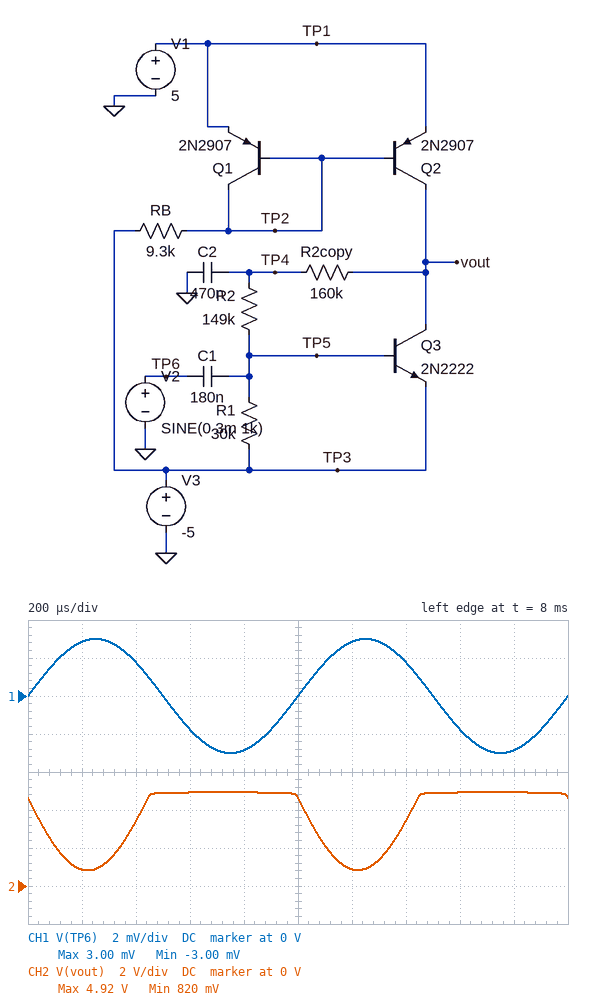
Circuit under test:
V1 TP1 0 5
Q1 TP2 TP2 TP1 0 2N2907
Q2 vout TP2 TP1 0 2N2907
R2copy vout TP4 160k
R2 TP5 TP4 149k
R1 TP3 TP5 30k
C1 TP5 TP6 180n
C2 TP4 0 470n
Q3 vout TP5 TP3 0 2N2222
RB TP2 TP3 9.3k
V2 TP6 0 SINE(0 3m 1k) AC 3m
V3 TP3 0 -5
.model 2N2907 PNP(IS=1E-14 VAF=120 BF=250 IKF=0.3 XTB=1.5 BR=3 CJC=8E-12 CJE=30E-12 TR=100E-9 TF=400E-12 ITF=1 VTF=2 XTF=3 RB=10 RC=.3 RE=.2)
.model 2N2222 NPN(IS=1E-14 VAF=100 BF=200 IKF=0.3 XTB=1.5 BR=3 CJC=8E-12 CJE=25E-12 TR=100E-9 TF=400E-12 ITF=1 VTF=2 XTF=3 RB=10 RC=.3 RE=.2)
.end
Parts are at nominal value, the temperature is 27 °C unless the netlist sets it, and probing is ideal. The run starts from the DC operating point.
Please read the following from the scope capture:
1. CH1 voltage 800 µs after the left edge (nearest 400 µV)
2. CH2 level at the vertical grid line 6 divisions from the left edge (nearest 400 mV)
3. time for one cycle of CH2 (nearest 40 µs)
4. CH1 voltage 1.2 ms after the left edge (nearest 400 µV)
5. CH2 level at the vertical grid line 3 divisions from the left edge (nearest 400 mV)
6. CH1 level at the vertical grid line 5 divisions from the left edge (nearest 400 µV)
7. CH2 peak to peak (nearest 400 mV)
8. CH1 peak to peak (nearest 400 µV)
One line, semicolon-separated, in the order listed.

-2.8 mV; 800 mV; 1.00 ms; 2.8 mV; 4.8 V; 0 V; 4.0 V; 6.0 mV
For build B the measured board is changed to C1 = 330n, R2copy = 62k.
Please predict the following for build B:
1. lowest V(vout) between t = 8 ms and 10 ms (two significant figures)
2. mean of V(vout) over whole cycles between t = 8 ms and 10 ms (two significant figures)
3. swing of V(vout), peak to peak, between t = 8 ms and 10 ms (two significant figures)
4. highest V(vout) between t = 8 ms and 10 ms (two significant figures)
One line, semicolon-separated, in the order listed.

-2.1 V; 1.3 V; 6.8 V; 4.6 V
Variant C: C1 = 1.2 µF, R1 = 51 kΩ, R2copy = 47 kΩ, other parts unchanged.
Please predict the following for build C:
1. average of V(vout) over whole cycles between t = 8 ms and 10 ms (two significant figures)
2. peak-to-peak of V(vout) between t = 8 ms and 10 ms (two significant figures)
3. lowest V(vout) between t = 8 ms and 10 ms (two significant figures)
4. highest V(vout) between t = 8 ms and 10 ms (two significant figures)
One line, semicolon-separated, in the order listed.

-940 mV; 6.0 V; -4.0 V; 2.0 V
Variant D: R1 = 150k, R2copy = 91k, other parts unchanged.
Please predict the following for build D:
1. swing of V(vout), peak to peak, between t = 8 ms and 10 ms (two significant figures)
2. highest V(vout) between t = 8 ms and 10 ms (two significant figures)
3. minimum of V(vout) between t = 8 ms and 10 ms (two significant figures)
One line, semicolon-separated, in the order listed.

6.5 V; 1.7 V; -4.9 V
